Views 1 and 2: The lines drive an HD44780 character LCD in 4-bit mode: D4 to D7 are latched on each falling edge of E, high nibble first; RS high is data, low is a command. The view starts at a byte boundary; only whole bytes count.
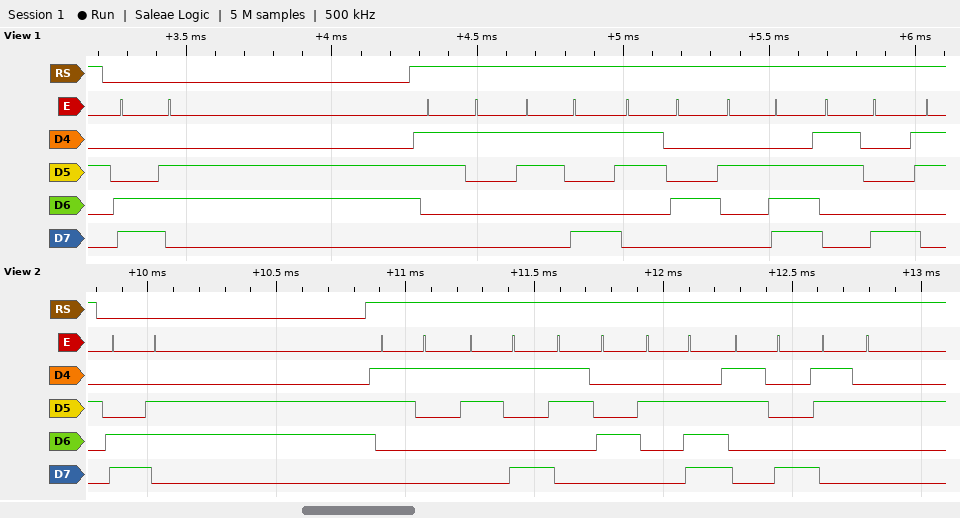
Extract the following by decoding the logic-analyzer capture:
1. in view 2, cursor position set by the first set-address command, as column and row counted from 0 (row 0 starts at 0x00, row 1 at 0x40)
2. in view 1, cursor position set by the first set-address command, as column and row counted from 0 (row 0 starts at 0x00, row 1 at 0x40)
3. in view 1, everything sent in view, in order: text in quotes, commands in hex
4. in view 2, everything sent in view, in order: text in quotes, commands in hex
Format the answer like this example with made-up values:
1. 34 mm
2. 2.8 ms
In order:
1. column 6, row 1
2. column 6, row 1
3. 0xC6 "194.8"
4. 0xC6 "194.82"
